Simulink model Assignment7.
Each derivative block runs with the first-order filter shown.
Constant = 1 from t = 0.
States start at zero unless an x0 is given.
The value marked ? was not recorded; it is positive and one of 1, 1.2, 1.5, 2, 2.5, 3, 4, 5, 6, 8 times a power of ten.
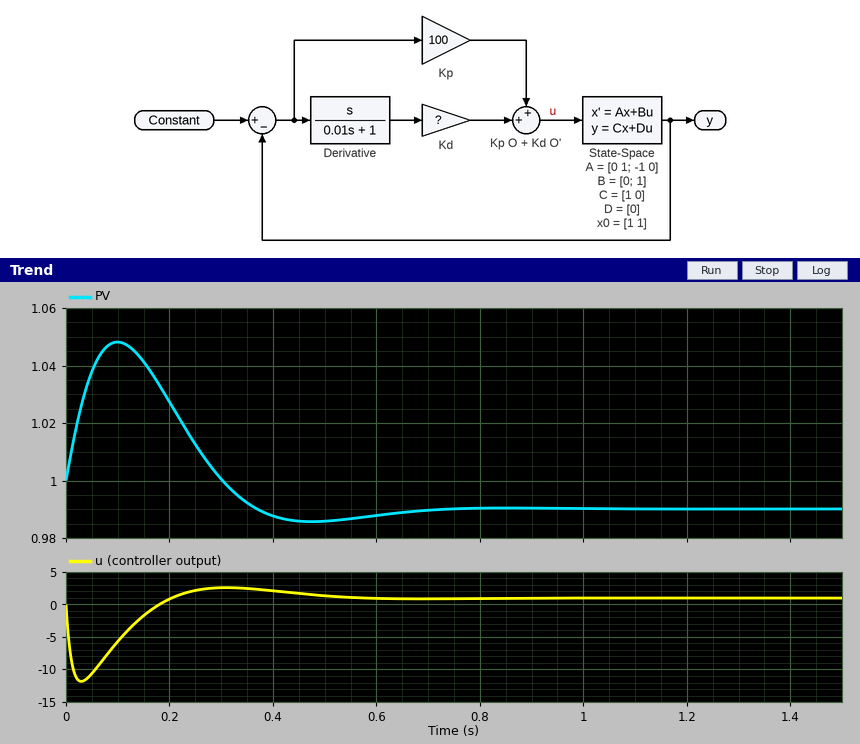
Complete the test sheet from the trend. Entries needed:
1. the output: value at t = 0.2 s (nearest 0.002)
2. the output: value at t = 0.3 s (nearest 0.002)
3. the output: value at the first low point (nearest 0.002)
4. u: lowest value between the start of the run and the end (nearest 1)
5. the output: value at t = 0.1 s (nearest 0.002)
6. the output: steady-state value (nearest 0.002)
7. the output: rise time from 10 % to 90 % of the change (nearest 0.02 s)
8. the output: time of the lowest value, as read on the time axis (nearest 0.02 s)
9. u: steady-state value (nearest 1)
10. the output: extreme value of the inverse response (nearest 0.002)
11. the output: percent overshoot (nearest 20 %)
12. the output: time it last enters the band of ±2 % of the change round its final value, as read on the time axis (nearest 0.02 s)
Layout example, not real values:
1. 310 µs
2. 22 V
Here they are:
1. 1.028
2. 1.000
3. 0.986
4. -12
5. 1.048
6. 0.990
7. 0.06 s
8. 0.48 s
9. 1
10. 1.048
11. 40 %
12. 0.96 s
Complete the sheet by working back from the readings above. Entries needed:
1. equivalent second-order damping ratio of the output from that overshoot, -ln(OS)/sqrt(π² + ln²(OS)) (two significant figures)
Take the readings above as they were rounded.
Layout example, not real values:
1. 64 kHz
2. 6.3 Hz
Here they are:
1. 0.28
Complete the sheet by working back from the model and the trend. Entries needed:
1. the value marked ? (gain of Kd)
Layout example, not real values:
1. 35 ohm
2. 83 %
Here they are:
1. 12
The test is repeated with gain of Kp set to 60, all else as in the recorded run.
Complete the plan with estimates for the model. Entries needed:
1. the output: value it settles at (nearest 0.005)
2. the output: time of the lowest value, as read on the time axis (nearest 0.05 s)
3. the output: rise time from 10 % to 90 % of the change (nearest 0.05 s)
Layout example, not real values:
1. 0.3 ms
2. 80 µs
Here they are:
1. 0.985
2. 0.75 s
3. 0.15 s
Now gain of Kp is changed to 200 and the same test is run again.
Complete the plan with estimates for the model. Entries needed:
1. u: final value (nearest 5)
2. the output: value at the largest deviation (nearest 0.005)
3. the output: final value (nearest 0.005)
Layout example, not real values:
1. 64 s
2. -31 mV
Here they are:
1. 0
2. 1.040
3. 0.995
